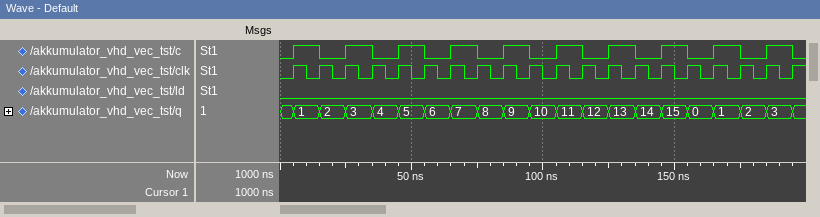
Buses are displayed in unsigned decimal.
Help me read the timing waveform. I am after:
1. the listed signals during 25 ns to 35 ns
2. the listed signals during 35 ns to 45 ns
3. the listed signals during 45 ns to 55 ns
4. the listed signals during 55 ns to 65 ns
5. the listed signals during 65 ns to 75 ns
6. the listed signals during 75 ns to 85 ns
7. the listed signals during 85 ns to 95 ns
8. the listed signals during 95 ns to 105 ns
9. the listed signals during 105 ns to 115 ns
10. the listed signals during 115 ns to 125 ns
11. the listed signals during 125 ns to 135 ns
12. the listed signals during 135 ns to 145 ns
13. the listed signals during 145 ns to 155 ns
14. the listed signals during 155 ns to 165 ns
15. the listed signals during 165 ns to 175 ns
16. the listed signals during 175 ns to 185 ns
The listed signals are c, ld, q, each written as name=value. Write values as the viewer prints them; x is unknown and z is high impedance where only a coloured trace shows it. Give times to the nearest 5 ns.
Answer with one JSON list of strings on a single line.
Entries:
["c=1, ld=0, q=3", "c=0, ld=0, q=4", "c=1, ld=0, q=5", "c=0, ld=0, q=6", "c=1, ld=0, q=7", "c=0, ld=0, q=8", "c=1, ld=0, q=9", "c=0, ld=0, q=10", "c=1, ld=0, q=11", "c=0, ld=0, q=12", "c=1, ld=0, q=13", "c=0, ld=0, q=14", "c=1, ld=0, q=15", "c=0, ld=0, q=0", "c=1, ld=0, q=1", "c=0, ld=0, q=2"]
